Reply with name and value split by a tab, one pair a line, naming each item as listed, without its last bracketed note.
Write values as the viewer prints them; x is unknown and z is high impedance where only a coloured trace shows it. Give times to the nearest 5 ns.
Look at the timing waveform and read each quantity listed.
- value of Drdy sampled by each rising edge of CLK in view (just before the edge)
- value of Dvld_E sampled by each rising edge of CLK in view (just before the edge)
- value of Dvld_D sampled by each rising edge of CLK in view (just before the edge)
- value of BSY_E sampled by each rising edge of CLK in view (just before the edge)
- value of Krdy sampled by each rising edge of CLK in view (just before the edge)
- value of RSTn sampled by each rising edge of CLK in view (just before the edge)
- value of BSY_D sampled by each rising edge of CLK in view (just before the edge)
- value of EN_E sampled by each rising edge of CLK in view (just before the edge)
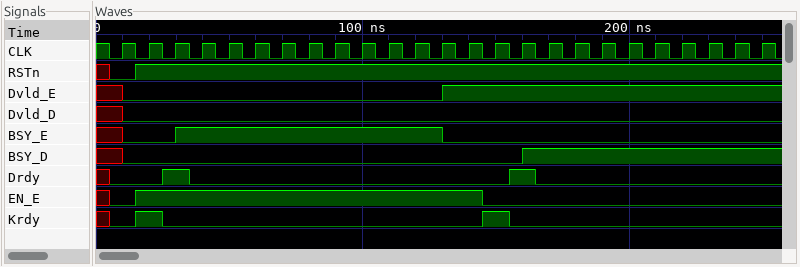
value of Drdy sampled by each rising edge of CLK in view	0 0 1 0 0 0 0 0 0 0 0 0 0 0 0 1 0 0 0 0 0 0 0 0 0
value of Dvld_E sampled by each rising edge of CLK in view	x 0 0 0 0 0 0 0 0 0 0 0 0 1 1 1 1 1 1 1 1 1 1 1 1
value of Dvld_D sampled by each rising edge of CLK in view	x 0 0 0 0 0 0 0 0 0 0 0 0 0 0 0 0 0 0 0 0 0 0 0 0
value of BSY_E sampled by each rising edge of CLK in view	x 0 0 1 1 1 1 1 1 1 1 1 1 0 0 0 0 0 0 0 0 0 0 0 0
value of Krdy sampled by each rising edge of CLK in view	0 1 0 0 0 0 0 0 0 0 0 0 0 0 1 0 0 0 0 0 0 0 0 0 0
value of RSTn sampled by each rising edge of CLK in view	0 1 1 1 1 1 1 1 1 1 1 1 1 1 1 1 1 1 1 1 1 1 1 1 1
value of BSY_D sampled by each rising edge of CLK in view	x 0 0 0 0 0 0 0 0 0 0 0 0 0 0 0 1 1 1 1 1 1 1 1 1
value of EN_E sampled by each rising edge of CLK in view	0 1 1 1 1 1 1 1 1 1 1 1 1 1 0 0 0 0 0 0 0 0 0 0 0
